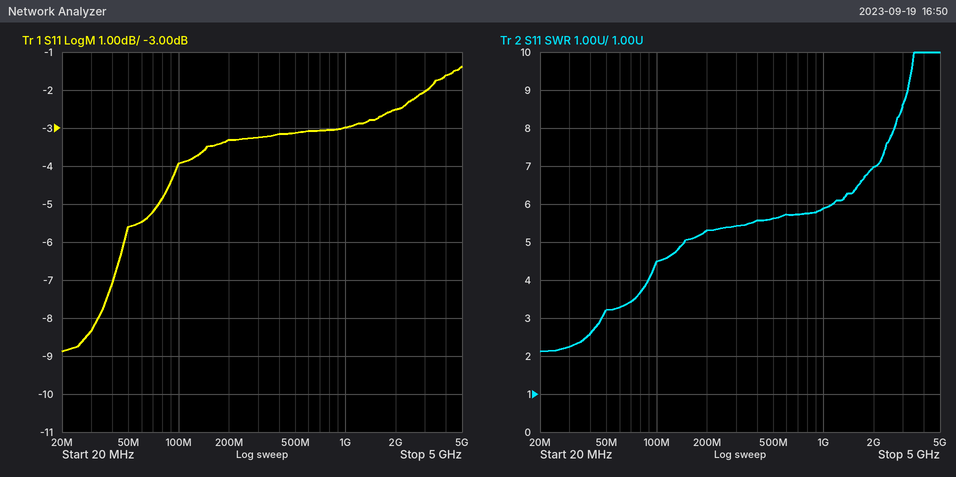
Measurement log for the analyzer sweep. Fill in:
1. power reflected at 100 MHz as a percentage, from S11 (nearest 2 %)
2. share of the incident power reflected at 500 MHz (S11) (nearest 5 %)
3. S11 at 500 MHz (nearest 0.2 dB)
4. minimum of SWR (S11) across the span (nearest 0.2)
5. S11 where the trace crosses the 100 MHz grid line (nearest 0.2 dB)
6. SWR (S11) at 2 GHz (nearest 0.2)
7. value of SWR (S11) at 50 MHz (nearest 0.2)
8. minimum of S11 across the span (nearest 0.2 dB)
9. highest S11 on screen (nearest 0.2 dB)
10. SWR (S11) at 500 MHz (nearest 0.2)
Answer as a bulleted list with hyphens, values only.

- 40 %
- 50 %
- -3.2 dB
- 2.2
- -4.0 dB
- 7.0
- 3.2
- -8.8 dB
- -1.4 dB
- 5.6
